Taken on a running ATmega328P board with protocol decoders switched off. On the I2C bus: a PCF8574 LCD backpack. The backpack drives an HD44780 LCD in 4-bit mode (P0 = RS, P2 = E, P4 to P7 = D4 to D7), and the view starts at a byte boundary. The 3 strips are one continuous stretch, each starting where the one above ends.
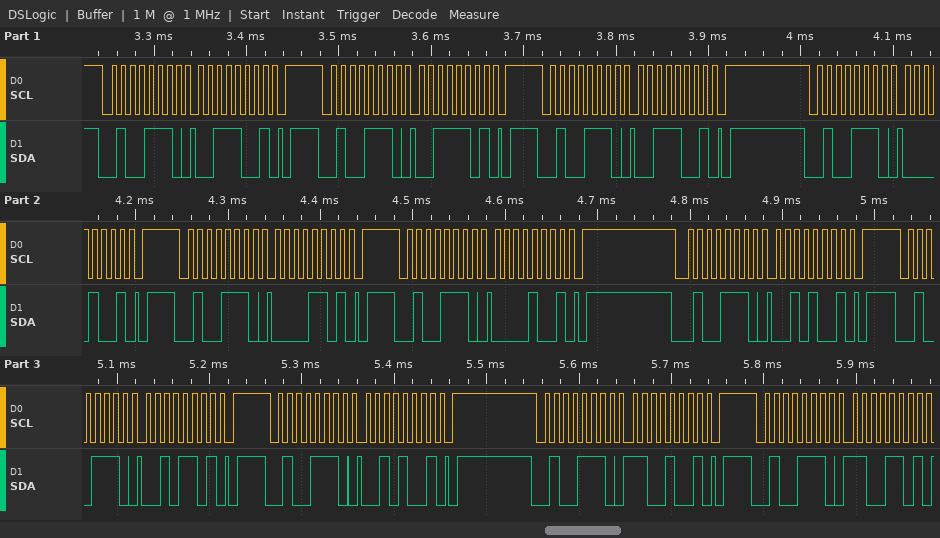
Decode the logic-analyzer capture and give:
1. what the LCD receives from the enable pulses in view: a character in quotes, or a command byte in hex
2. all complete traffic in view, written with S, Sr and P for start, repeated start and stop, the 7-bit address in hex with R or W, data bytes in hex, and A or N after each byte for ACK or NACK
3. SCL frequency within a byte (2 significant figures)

'0'
S 27W A 39 A P S 27W A 3D A P S 27W A 39 A P S 27W A 09 A P S 27W A 0D A P S 27W A 09 A P S 27W A 29 A P S 27W A 2D A P S 27W A 29 A P S 27W A C9 A P S 27W A CD A
100 kHz
